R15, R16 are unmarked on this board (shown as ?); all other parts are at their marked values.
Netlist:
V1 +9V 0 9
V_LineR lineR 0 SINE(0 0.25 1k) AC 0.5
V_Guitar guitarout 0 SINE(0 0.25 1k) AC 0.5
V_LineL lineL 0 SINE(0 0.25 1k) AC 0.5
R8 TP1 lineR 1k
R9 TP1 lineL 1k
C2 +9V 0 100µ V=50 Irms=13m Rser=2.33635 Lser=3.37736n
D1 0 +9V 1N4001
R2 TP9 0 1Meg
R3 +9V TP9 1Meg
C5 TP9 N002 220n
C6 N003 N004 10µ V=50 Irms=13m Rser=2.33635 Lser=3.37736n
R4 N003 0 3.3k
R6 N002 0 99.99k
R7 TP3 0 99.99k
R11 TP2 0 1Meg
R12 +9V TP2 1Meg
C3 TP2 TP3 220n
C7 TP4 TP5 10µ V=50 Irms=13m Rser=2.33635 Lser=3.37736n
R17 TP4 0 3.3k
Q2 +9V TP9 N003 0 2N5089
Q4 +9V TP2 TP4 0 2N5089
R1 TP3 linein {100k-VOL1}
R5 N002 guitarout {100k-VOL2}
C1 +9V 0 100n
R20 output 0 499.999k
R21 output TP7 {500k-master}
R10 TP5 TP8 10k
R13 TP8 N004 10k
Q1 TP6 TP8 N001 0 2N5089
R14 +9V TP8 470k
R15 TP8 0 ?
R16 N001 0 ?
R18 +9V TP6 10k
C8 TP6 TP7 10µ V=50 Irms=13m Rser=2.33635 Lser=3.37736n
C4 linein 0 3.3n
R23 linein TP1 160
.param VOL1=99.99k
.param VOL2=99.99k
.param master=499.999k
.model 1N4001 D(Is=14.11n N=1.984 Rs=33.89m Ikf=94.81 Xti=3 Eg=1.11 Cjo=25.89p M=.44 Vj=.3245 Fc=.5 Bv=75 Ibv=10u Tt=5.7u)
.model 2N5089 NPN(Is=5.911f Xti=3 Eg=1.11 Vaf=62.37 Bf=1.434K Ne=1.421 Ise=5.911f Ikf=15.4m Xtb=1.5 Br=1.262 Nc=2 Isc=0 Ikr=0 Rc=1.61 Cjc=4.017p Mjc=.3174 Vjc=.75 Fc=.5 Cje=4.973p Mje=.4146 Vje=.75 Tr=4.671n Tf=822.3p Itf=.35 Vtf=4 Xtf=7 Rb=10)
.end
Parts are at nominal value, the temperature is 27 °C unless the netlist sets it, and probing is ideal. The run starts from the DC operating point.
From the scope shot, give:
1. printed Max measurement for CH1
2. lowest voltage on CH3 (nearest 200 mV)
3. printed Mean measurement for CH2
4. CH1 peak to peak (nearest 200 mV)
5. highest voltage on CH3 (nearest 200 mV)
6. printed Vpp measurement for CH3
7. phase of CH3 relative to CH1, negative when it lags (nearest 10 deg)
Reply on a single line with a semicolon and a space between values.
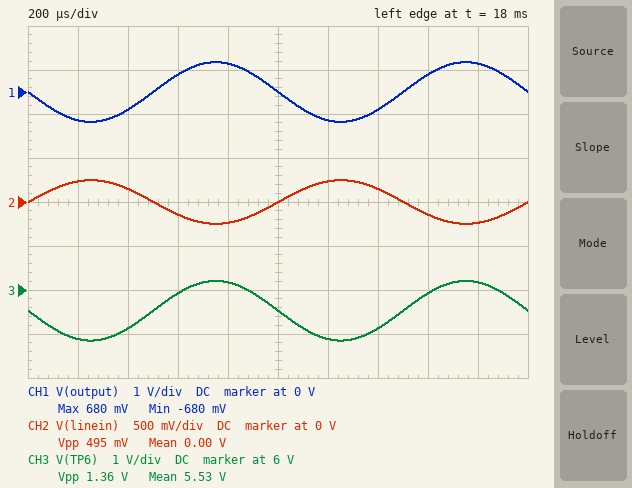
680 mV; 4.8 V; 0.00 V; 1.4 V; 6.2 V; 1.36 V; 0 deg
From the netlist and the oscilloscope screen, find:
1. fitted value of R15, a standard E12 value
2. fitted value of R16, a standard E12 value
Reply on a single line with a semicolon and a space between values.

120 kΩ; 3.3 kΩ
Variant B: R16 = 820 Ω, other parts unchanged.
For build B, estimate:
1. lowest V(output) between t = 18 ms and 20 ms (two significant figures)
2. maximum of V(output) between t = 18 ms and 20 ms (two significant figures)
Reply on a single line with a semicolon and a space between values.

-29 mV; 2.5 V
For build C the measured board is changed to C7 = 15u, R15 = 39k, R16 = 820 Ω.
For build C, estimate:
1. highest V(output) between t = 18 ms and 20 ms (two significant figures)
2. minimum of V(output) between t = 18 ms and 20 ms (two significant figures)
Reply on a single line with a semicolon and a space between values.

940 mV; -2.2 V
